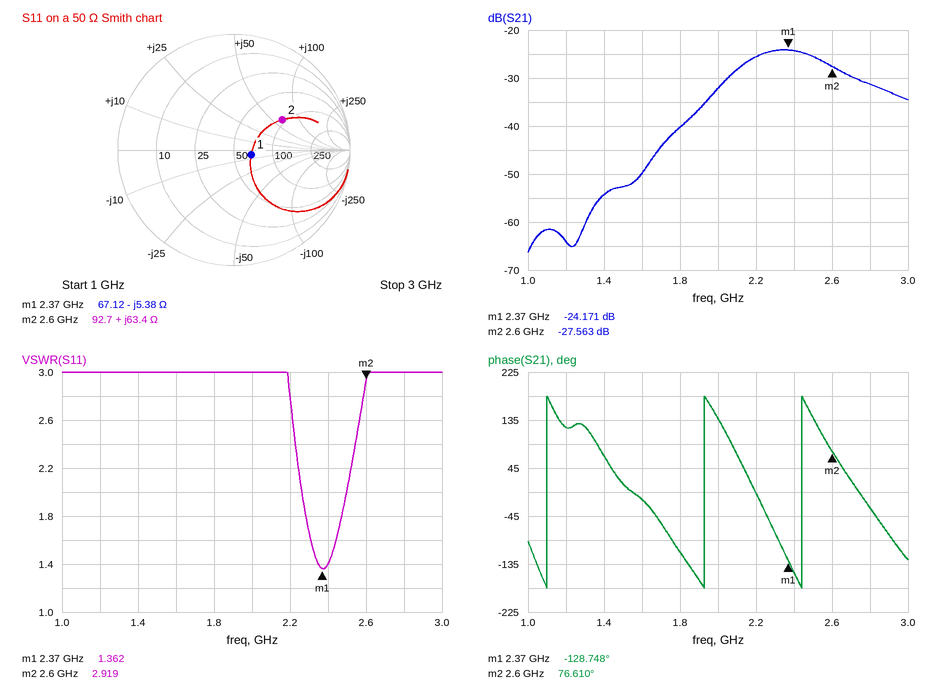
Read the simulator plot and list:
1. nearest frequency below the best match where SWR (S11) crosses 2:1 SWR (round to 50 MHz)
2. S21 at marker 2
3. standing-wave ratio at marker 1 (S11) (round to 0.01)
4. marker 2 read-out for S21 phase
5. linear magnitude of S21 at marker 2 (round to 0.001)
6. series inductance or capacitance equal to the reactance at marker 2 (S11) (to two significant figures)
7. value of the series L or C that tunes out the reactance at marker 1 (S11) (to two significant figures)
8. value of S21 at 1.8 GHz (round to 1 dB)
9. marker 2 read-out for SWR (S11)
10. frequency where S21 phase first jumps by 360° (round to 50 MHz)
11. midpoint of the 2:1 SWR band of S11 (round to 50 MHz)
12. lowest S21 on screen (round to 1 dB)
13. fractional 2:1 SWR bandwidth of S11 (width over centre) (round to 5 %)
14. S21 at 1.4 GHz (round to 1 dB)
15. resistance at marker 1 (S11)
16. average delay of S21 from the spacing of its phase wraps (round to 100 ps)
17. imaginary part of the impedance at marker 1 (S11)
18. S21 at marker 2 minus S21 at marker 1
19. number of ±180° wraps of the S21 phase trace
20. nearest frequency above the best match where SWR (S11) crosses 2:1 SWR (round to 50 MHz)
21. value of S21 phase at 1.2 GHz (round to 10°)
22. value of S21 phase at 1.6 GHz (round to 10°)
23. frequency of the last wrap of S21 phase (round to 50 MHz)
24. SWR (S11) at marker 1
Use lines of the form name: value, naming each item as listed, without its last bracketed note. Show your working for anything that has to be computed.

nearest frequency below the best match where SWR (S11) crosses 2:1 SWR: 2.25 GHz
S21 at marker 2: -27.563 dB
standing-wave ratio at marker 1 (S11): 1.36
marker 2 read-out for S21 phase: 76.610°
linear magnitude of S21 at marker 2: 10^(-27.563/20) ≈ 0.042
series inductance or capacitance equal to the reactance at marker 2 (S11): L = 63.4 Ω/(2π × 2.6 GHz) ≈ 3.9 nH
value of the series L or C that tunes out the reactance at marker 1 (S11): L = 5.38 Ω/(2π × 2.37 GHz) ≈ 361 pH, so 360 pH to two significant figures
value of S21 at 1.8 GHz: -40 dB
marker 2 read-out for SWR: 2.919
frequency where S21 phase first jumps by 360°: 1.10 GHz
midpoint of the 2:1 SWR band of S11: 2.40 GHz
lowest S21 on screen: -66 dB
fractional 2:1 SWR bandwidth of S11 (width over centre): 250 MHz / 2.375 GHz ≈ 10 %
S21 at 1.4 GHz: -54 dB
resistance at marker 1: 67.12 Ω
average delay of S21 from the spacing of its phase wraps: 2 cycles / (2.45 GHz − 1.10 GHz) ≈ 1.5 ns
imaginary part of the impedance at marker 1: -5.38 Ω
S21 at marker 2 minus S21 at marker 1: -27.563 − (-24.171) = -3.392 dB
number of ±180° wraps of the S21 phase trace: 3
nearest frequency above the best match where SWR (S11) crosses 2:1 SWR: 2.50 GHz
value of S21 phase at 1.2 GHz: 120°
value of S21 phase at 1.6 GHz: -10°
frequency of the last wrap of S21 phase: 2.45 GHz
SWR (S11) at marker 1: 1.362
